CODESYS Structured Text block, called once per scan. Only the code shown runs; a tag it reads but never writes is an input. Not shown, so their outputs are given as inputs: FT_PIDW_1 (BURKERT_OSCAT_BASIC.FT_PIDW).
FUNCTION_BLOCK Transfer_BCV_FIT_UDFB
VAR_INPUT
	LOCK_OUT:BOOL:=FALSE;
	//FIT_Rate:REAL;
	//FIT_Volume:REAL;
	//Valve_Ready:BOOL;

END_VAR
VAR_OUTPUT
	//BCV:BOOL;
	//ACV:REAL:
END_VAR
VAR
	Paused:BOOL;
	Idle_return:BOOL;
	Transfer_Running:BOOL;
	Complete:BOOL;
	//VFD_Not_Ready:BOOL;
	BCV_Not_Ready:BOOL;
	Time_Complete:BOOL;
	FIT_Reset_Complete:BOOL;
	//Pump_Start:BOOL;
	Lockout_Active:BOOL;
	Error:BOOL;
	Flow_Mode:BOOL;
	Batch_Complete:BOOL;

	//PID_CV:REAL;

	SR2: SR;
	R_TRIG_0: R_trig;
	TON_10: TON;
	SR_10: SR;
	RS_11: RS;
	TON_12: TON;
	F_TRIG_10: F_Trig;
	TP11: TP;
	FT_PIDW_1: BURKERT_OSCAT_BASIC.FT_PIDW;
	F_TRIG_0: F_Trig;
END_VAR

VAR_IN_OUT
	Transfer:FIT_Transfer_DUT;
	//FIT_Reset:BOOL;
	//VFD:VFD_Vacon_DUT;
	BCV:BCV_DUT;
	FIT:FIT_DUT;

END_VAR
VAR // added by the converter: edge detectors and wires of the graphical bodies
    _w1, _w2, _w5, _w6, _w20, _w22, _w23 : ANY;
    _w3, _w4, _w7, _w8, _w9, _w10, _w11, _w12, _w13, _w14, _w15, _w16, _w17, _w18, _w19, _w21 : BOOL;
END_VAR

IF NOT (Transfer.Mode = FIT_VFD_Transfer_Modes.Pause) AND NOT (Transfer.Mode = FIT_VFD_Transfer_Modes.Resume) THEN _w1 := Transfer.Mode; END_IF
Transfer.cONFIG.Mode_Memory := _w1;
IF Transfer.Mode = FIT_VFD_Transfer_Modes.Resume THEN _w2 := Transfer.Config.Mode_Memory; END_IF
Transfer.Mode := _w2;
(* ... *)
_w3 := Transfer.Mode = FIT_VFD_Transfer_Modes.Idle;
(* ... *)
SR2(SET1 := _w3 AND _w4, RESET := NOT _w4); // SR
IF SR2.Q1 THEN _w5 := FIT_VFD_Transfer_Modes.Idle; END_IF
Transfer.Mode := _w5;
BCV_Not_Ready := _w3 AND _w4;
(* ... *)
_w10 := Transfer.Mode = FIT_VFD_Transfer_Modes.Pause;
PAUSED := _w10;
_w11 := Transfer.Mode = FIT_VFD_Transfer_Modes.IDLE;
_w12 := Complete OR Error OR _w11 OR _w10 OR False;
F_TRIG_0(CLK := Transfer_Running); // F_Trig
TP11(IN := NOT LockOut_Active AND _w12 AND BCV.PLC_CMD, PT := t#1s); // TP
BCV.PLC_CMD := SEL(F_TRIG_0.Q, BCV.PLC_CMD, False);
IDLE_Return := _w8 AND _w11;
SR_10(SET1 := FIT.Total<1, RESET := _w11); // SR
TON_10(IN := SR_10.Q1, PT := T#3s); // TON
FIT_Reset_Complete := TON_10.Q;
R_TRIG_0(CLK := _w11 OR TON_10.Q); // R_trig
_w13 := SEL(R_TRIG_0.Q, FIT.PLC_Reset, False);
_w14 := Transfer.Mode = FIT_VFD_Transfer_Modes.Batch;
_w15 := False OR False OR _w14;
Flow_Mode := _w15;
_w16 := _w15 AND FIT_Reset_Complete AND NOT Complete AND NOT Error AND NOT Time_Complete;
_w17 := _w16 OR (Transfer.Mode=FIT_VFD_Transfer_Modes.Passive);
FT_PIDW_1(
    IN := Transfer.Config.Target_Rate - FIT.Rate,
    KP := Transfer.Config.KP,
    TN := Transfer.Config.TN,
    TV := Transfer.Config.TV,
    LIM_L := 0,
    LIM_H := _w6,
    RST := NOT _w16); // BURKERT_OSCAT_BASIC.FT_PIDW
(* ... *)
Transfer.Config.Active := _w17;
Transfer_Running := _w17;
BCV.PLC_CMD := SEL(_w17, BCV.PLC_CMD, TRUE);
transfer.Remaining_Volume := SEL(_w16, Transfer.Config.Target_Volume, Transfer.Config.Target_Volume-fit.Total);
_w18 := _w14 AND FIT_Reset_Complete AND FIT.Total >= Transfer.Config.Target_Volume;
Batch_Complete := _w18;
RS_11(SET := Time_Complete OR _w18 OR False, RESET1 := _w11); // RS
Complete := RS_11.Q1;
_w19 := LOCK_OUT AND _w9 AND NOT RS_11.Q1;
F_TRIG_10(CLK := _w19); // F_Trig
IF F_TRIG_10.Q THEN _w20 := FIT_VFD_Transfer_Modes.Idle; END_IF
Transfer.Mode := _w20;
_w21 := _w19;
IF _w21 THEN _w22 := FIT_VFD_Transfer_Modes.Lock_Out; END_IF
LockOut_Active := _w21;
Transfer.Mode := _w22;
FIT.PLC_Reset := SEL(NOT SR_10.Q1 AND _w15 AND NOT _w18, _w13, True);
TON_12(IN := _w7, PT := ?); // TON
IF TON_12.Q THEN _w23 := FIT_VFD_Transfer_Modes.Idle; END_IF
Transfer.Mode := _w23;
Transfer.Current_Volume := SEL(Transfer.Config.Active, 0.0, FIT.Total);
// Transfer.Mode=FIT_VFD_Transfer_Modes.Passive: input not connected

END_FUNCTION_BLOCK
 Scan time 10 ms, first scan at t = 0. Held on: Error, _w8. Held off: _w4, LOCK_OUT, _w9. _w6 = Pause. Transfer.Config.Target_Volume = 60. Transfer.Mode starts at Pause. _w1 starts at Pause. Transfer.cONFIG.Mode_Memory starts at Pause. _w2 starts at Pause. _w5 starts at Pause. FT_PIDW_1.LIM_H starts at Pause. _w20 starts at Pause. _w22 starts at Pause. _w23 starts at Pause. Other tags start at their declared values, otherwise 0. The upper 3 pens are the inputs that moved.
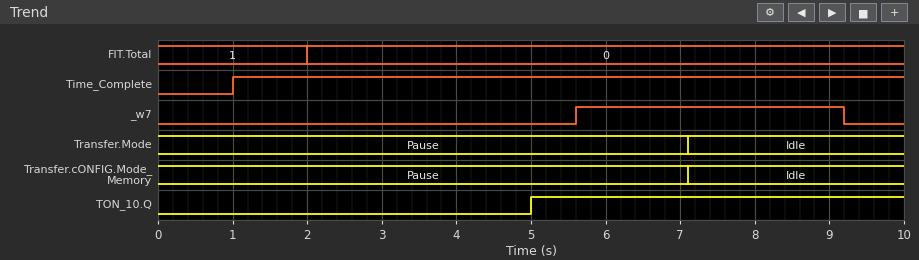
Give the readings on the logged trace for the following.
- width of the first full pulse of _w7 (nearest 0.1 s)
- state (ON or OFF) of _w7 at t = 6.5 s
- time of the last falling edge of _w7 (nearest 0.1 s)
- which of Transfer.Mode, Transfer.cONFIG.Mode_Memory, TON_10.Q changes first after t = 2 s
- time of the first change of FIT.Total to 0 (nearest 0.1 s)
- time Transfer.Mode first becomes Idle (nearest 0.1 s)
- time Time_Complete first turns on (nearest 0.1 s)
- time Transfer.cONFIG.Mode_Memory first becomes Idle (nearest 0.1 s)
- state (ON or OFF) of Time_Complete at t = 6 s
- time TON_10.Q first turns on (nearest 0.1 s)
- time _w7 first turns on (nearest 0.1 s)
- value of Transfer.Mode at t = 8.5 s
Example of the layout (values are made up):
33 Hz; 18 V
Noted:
3.6 s; ON; 9.2 s; TON_10.Q; 2.0 s; 7.1 s; 1.0 s; 7.1 s; ON; 5.0 s; 5.6 s; Idle
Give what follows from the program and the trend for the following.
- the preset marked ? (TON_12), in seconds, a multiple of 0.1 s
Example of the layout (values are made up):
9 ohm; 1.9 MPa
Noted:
1.5 s
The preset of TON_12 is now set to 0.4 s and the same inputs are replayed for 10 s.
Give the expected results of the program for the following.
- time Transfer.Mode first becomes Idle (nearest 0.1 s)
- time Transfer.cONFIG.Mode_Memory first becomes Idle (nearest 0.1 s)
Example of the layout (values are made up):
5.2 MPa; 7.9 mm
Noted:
6.0 s; 6.0 s
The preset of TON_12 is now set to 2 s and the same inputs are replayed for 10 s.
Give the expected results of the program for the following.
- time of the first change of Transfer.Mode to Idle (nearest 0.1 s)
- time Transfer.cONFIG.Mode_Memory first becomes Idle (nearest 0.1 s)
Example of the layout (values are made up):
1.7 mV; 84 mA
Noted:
7.6 s; 7.6 s
